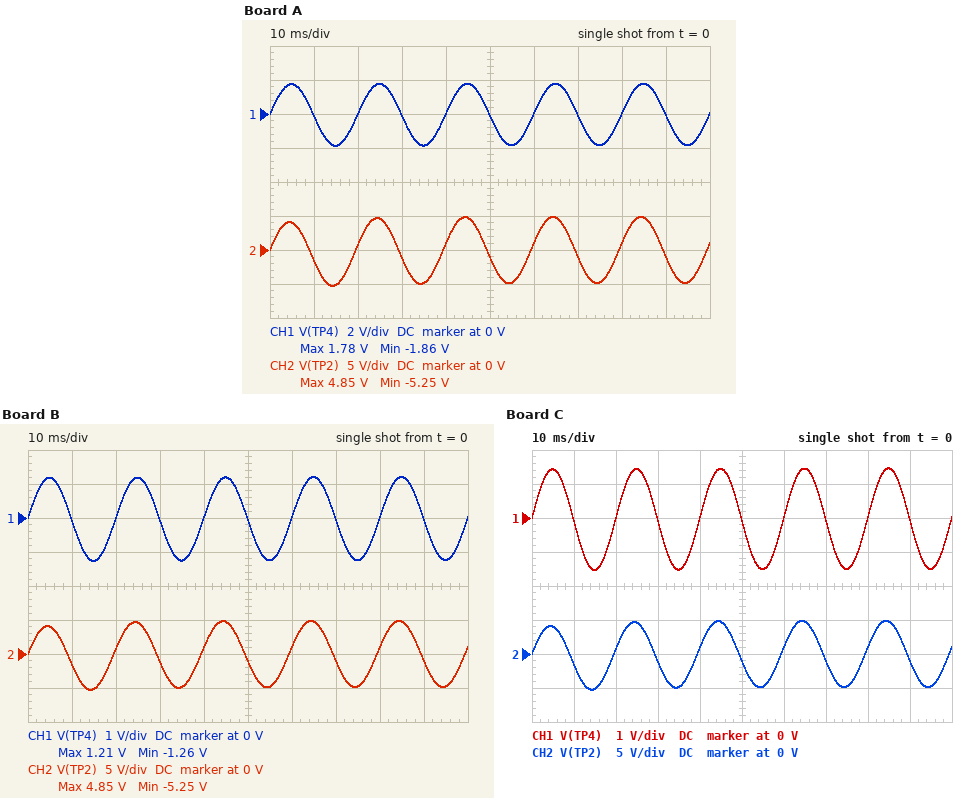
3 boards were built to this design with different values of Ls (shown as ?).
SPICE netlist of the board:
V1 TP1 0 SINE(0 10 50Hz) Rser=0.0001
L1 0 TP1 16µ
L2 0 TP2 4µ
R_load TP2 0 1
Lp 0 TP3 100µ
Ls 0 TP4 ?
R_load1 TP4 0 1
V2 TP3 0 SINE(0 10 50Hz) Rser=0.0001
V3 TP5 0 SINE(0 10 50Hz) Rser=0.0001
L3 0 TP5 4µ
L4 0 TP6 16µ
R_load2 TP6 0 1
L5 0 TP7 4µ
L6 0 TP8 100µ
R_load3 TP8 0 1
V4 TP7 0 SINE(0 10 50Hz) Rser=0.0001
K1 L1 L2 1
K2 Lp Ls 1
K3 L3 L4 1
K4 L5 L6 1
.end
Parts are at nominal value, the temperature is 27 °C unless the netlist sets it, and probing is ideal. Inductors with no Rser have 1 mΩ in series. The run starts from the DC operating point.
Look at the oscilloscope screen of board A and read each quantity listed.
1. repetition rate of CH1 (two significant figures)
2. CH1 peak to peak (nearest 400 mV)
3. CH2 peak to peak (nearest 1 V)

50 Hz
3.6 V
10 V
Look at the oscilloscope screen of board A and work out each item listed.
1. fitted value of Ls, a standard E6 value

3.3 µH
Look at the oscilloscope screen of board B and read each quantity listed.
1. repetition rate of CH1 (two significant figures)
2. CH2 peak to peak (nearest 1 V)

50 Hz
10 V
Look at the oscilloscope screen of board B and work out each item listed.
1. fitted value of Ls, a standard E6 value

1.5 µH
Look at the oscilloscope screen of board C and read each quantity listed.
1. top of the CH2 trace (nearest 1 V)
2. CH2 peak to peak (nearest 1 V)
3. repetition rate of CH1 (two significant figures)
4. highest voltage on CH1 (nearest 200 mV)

5 V
10 V
50 Hz
1.4 V
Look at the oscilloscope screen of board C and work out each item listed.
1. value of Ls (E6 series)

2.2 µH
